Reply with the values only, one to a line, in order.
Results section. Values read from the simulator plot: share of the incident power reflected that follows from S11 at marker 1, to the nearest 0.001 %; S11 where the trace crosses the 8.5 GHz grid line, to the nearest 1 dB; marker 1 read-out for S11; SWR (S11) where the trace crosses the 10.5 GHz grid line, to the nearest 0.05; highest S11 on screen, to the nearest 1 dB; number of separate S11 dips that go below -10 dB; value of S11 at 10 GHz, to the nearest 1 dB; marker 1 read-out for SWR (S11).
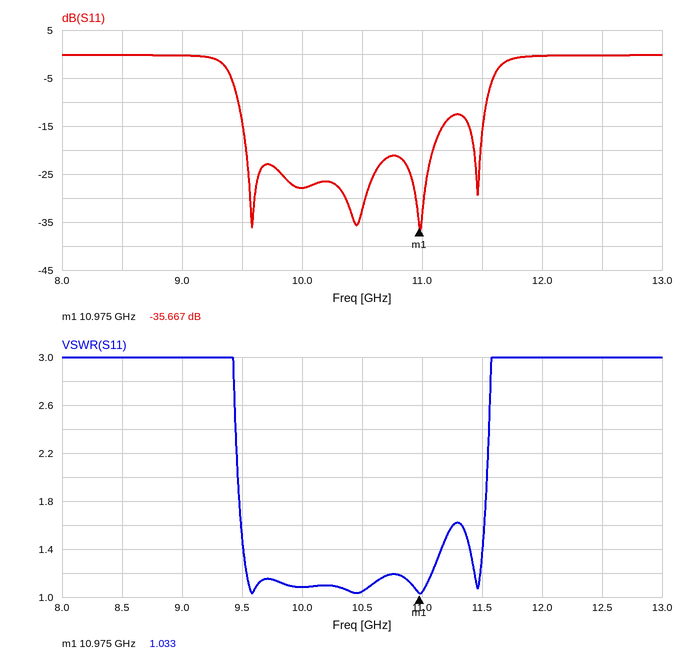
0.027 %
0 dB
-35.667 dB
1.05
0 dB
4
-28 dB
1.033
